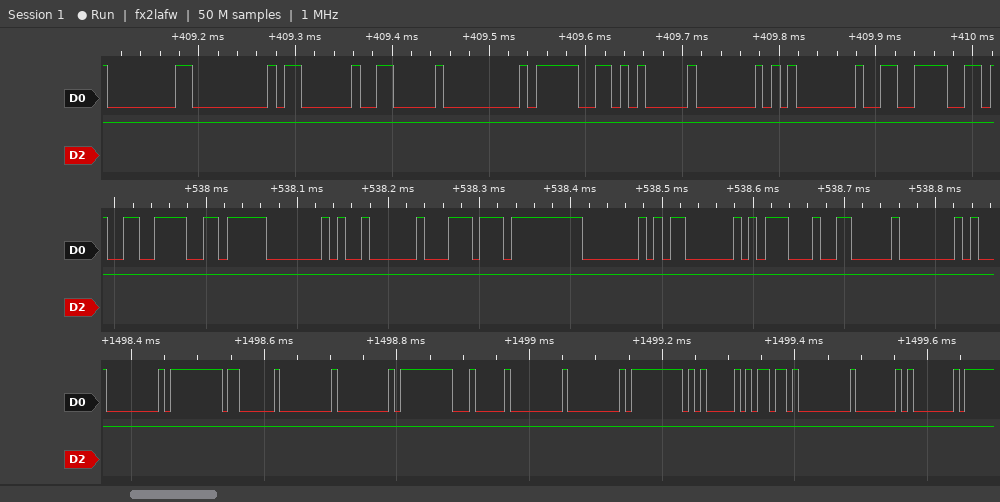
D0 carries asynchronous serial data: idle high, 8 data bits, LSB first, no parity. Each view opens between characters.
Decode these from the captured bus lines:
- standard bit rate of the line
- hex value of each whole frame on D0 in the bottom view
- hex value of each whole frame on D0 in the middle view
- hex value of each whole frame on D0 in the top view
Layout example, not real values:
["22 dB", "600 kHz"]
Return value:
["115200 baud", "00, FF, 03, 00, 00, FF, 04, 00, 00, FF, 05, 6D, 00, 40, 40", "E6, F6, 40, 02, DC, FF, 40, 03, 1D, 06, 40", "80, 00, 03, 06, 00, 9F, 05, 40, 01, E6"]
